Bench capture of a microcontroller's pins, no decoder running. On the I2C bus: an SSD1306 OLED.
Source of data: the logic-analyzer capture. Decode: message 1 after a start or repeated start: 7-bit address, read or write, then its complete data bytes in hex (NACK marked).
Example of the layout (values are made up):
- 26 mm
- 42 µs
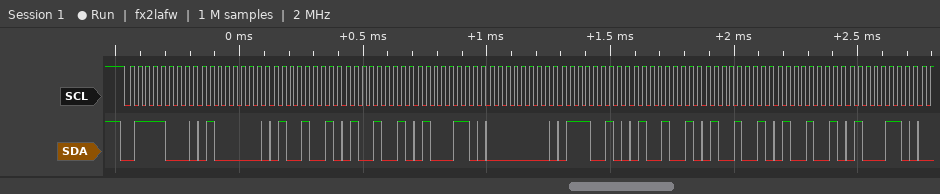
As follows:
- 0x3C write: 40 49 49 46 00 72 49 49 49 46
